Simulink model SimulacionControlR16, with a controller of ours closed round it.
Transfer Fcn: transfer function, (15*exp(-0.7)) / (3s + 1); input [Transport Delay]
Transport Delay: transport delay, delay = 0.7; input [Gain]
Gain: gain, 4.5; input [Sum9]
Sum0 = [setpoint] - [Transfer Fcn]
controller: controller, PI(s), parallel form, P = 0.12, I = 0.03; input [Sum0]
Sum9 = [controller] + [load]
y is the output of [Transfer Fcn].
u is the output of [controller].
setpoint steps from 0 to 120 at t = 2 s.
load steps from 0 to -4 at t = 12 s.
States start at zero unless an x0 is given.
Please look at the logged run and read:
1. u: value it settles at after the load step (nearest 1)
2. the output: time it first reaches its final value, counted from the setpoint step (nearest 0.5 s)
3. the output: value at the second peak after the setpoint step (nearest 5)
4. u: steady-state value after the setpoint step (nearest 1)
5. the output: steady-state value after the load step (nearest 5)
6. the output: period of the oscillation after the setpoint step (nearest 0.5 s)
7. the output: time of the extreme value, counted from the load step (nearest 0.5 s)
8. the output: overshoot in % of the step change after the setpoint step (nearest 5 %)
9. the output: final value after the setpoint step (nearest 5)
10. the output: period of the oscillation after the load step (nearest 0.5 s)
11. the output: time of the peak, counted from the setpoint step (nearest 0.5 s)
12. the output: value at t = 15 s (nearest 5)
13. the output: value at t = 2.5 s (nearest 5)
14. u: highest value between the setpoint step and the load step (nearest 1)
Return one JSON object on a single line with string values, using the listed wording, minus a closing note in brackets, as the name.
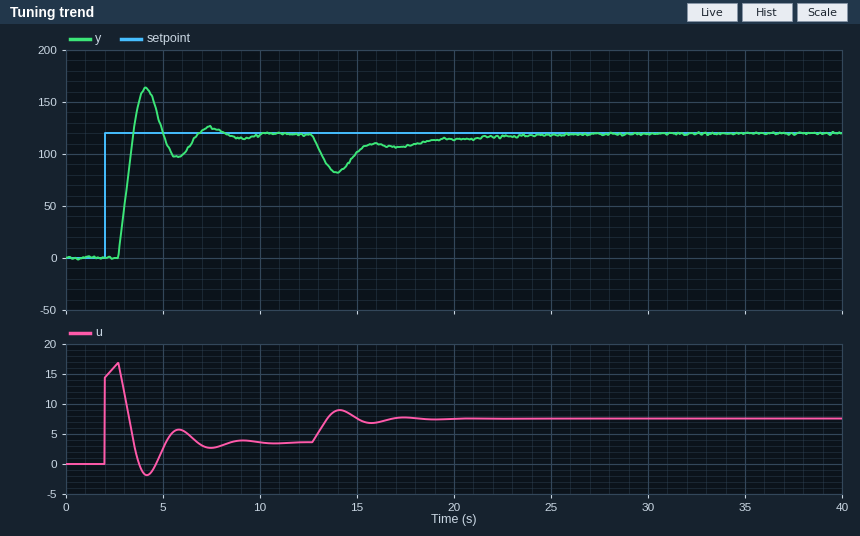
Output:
{"u: value it settles at after the load step": "8", "the output: time it first reaches its final value, counted from the setpoint step": "1.5 s", "the output: value at the second peak after the setpoint step": "125", "u: steady-state value after the setpoint step": "4", "the output: steady-state value after the load step": "120", "the output: period of the oscillation after the setpoint step": "3.5 s", "the output: time of the extreme value, counted from the load step": "2.0 s", "the output: overshoot in % of the step change after the setpoint step": "35 %", "the output: final value after the setpoint step": "120", "the output: period of the oscillation after the load step": "3.0 s", "the output: time of the peak, counted from the setpoint step": "2.0 s", "the output: value at t = 15 s": "100", "the output: value at t = 2.5 s": "0", "u: highest value between the setpoint step and the load step": "17"}
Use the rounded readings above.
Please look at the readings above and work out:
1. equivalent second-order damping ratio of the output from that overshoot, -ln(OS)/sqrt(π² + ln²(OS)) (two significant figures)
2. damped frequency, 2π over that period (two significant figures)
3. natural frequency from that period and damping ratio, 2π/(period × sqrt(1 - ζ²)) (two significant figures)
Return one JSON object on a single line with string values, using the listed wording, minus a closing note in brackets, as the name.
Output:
{"equivalent second-order damping ratio of the output from that overshoot, -ln(OS)/sqrt(π² + ln²(OS))": "0.32", "damped frequency, 2π over that period": "1.8 rad/s", "natural frequency from that period and damping ratio, 2π/(period × sqrt(1 - ζ²))": "1.9 rad/s"}
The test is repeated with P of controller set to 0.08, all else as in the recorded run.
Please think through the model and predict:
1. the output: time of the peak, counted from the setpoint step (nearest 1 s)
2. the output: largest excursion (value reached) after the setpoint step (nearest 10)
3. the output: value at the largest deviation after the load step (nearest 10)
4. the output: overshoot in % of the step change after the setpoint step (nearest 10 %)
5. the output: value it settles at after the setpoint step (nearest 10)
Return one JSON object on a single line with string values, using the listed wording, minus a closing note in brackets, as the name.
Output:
{"the output: time of the peak, counted from the setpoint step": "3 s", "the output: largest excursion (value reached) after the setpoint step": "140", "the output: value at the largest deviation after the load step": "80", "the output: overshoot in % of the step change after the setpoint step": "20 %", "the output: value it settles at after the setpoint step": "120"}
